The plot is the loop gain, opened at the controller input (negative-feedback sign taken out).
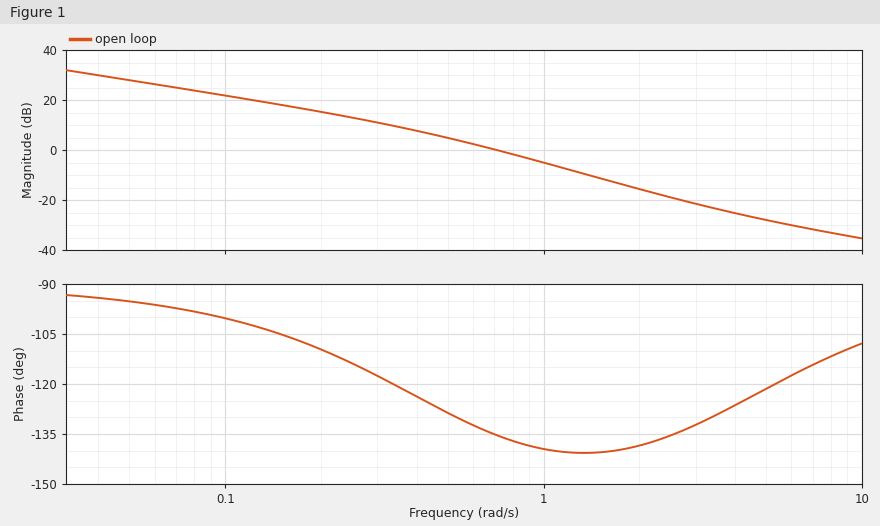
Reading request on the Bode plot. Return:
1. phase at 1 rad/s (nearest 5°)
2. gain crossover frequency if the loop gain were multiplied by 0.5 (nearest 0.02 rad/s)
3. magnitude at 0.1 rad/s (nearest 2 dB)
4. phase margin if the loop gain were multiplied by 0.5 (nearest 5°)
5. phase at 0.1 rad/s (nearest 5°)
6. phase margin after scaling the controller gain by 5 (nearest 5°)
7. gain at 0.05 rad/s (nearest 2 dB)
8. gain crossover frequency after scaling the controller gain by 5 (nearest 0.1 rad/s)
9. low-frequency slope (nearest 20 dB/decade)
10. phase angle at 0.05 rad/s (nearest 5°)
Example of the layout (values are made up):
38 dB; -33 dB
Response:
-140°; 0.46 rad/s; 22 dB; 55°; -100°; 40°; 28 dB; 1.8 rad/s; -20 dB/decade; -95°
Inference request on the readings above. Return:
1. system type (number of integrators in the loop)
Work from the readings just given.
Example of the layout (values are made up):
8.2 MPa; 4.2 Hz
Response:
1
